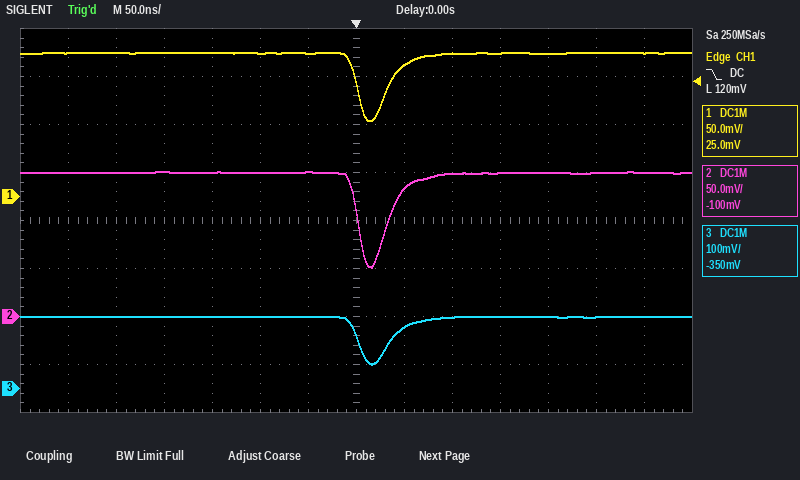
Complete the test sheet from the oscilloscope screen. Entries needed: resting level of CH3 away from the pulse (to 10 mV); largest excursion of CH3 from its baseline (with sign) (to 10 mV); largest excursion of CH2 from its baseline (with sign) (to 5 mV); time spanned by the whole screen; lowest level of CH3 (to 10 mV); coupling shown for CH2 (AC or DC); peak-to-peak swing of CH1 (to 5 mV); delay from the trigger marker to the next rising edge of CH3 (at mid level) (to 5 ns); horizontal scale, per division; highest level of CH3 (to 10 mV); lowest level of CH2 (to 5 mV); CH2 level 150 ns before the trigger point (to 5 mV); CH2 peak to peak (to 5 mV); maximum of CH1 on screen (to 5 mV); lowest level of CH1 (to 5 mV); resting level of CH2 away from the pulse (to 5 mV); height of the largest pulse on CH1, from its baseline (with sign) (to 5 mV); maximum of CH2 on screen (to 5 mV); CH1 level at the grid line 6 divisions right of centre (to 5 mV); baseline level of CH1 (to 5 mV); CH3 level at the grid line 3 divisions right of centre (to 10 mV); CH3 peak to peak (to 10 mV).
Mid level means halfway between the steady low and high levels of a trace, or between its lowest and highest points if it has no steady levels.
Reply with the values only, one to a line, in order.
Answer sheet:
150 mV
-100 mV
-100 mV
700 ns
50 mV
DC
70 mV
35 ns
50 ns
150 mV
50 mV
150 mV
100 mV
150 mV
80 mV
150 mV
-70 mV
150 mV
150 mV
150 mV
150 mV
100 mV
